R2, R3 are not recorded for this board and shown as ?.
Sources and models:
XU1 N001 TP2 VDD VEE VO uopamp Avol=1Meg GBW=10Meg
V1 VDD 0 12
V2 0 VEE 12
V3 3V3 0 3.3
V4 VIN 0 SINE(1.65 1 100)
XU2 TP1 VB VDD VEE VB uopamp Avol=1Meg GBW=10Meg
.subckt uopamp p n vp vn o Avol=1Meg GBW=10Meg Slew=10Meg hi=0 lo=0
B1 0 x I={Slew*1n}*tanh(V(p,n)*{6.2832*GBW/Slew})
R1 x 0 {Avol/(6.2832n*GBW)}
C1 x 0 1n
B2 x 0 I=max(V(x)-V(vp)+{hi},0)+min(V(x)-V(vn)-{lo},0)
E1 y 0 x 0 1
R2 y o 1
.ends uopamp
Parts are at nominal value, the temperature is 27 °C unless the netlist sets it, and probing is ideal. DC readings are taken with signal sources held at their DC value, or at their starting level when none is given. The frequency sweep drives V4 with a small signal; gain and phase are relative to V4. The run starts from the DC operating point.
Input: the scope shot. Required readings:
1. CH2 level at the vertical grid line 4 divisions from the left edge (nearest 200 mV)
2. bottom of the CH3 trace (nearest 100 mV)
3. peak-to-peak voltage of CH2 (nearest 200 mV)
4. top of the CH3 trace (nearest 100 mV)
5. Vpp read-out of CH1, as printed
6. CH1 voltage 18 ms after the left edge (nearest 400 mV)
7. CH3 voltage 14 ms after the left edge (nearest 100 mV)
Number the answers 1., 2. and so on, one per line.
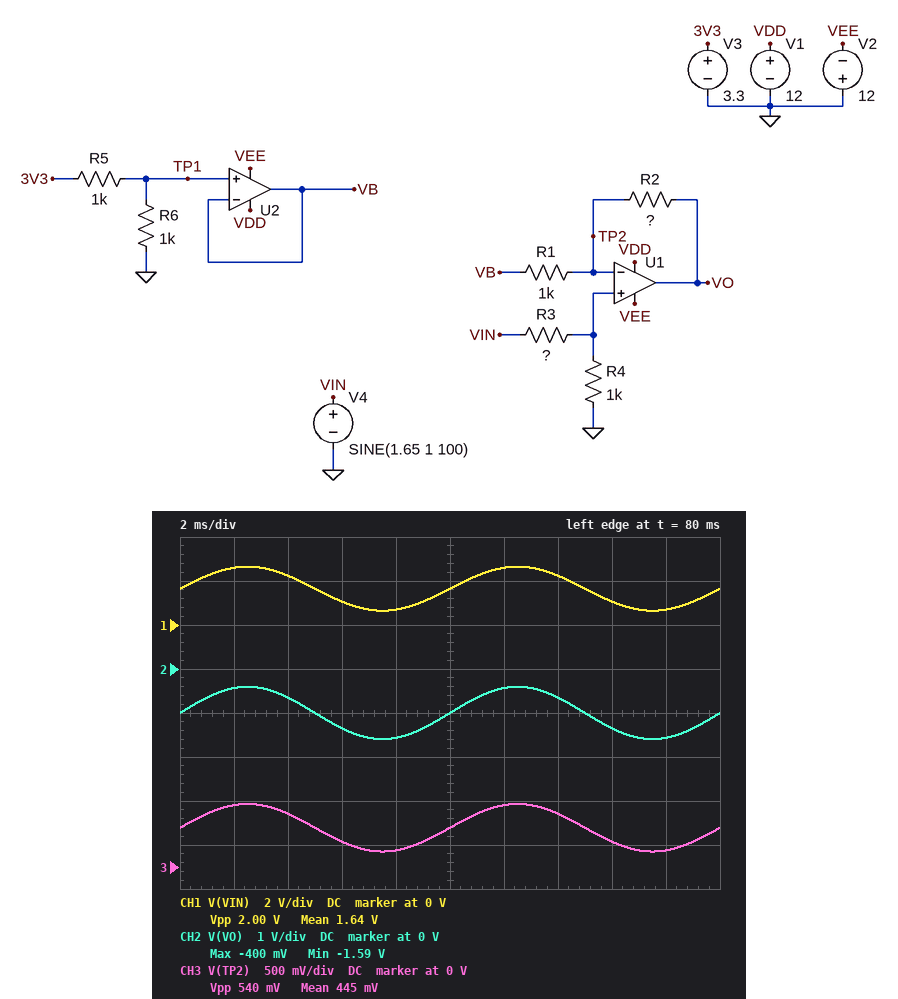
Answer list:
1. -1.6 V
2. 200 mV
3. 1.2 V
4. 700 mV
5. 2.00 V
6. 800 mV
7. 600 mV
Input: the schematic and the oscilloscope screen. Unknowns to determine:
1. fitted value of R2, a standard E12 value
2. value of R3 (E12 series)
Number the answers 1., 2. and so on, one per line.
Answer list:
1. 1.2 kΩ
2. 2.7 kΩ
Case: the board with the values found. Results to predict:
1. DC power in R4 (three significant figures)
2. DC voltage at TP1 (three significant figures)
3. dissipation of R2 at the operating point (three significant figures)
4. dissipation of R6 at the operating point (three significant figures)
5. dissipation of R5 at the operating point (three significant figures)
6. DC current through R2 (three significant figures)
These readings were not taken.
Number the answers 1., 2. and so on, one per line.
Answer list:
1. 199 µW
2. 1.65 V
3. 1.74 mW
4. 2.72 mW
5. 2.72 mW
6. 1.20 mA
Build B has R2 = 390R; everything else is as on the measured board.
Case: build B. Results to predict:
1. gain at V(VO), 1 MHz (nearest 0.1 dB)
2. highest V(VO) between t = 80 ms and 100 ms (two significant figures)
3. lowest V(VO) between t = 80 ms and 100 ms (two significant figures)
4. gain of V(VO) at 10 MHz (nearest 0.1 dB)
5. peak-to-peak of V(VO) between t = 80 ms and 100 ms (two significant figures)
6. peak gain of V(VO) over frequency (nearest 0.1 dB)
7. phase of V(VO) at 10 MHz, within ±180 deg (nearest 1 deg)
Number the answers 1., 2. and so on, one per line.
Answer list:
1. -8.6 dB
2. 350 mV
3. -400 mV
4. -13.2 dB
5. 750 mV
6. -8.5 dB
7. -54 deg
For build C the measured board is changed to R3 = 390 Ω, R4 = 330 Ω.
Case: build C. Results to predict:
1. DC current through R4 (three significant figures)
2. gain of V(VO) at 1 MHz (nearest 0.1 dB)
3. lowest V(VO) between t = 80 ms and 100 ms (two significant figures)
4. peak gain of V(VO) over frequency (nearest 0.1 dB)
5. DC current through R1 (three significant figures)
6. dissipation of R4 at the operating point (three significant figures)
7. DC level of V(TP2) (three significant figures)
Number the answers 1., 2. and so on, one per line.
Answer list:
1. 2.29 mA
2. -0.1 dB
3. -1.3 V
4. 0.1 dB
5. 894 µA
6. 1.73 mW
7. 756 mV
